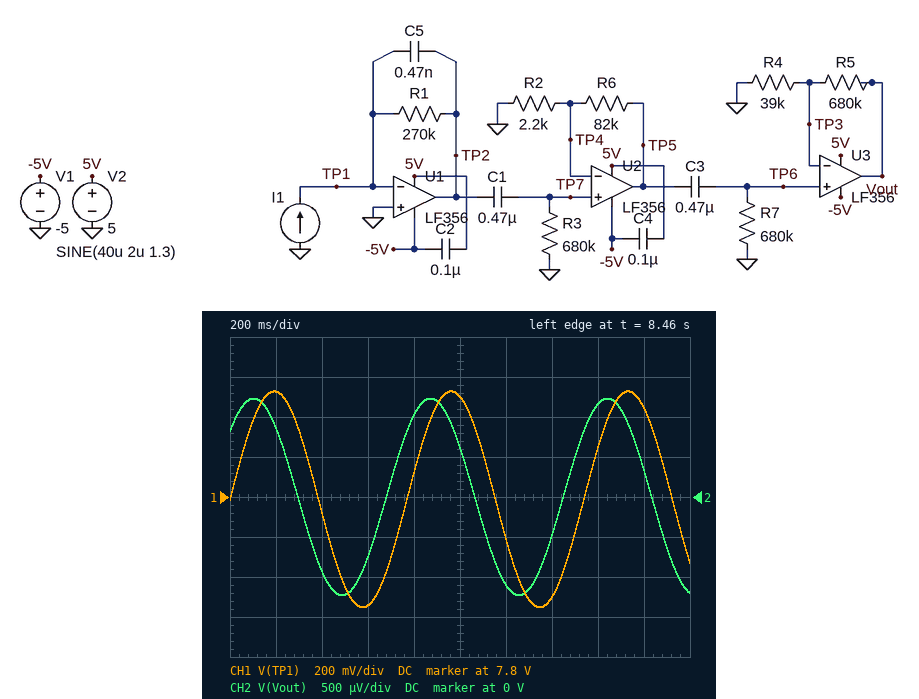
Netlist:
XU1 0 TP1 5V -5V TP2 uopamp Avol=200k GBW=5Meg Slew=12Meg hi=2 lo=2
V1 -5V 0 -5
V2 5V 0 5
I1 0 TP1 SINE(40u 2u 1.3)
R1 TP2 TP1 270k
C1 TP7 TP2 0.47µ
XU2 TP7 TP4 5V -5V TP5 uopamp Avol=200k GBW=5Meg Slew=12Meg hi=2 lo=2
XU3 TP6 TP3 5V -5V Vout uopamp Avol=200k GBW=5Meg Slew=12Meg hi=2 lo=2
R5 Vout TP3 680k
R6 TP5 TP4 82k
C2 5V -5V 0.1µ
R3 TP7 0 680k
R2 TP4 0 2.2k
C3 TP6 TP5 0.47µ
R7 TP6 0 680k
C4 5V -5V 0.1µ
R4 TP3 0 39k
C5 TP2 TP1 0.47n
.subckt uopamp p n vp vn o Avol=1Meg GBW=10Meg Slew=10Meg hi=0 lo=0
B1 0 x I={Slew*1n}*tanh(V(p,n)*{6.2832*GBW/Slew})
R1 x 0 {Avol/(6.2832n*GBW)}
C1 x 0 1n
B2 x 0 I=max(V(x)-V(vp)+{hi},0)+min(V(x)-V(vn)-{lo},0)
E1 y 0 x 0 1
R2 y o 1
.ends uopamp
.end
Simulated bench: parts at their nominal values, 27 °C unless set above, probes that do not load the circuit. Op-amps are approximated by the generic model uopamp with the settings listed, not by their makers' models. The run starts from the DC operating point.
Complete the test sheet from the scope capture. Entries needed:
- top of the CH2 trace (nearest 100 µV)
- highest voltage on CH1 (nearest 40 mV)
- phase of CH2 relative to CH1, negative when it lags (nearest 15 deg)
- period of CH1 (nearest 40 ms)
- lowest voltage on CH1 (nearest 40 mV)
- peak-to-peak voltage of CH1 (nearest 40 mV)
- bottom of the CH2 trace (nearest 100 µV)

1.2 mV
8.32 V
45 deg
760 ms
7.24 V
1.08 V
-1.2 mV
